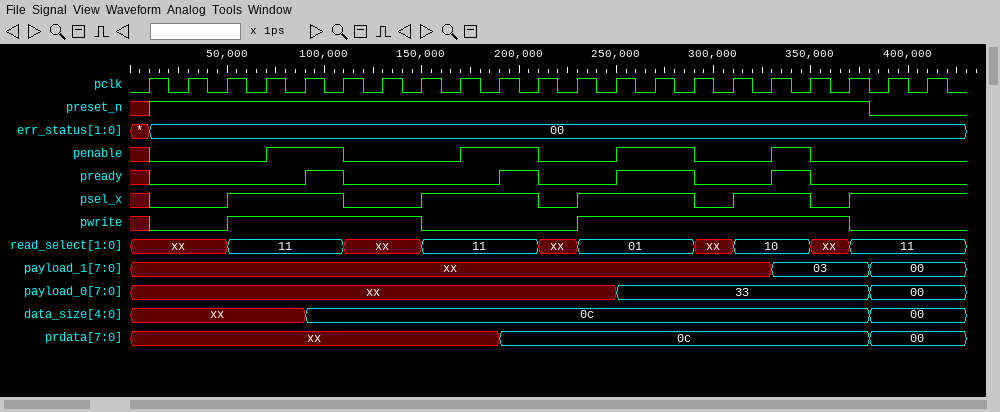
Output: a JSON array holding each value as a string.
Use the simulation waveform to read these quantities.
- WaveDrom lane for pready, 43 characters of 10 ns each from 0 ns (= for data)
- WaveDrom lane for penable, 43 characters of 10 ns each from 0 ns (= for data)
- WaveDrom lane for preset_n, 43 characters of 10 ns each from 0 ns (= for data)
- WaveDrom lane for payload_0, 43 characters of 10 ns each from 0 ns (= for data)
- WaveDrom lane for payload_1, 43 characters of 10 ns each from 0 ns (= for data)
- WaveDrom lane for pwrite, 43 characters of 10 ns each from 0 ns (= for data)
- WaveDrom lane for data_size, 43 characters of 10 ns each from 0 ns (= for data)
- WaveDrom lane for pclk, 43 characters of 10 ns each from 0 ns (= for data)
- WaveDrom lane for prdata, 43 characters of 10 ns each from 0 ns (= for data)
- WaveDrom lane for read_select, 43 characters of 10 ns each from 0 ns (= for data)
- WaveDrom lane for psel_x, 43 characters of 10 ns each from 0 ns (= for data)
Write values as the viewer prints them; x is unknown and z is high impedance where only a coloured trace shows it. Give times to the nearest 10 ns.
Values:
["{name: 'pready', wave: 'x0.......1.0.......1.0...1...0...1.0.......'}", "{name: 'penable', wave: 'x0.....1...0.....1...0...1...0...1.0.......'}", "{name: 'preset_n', wave: 'x1....................................0....'}", "{name: 'payload_0', wave: 'x........................=............=....', data: '33 00'}", "{name: 'payload_1', wave: 'x................................=....=....', data: '03 00'}", "{name: 'pwrite', wave: 'x0...1.........0.......1.............0.....'}", "{name: 'data_size', wave: 'x........=............................=....', data: '0c 00'}", "{name: 'pclk', wave: '0101010101010101010101010101010101010101010'}", "{name: 'prdata', wave: 'x..................=..................=....', data: '0c 00'}", "{name: 'read_select', wave: 'x....=.....x...=.....x.=.....x.=...x.=.....', data: '11 11 01 10 11'}", "{name: 'psel_x', wave: 'x0...1.....0...1.....0.1.....0.1...0.1.....'}"]
